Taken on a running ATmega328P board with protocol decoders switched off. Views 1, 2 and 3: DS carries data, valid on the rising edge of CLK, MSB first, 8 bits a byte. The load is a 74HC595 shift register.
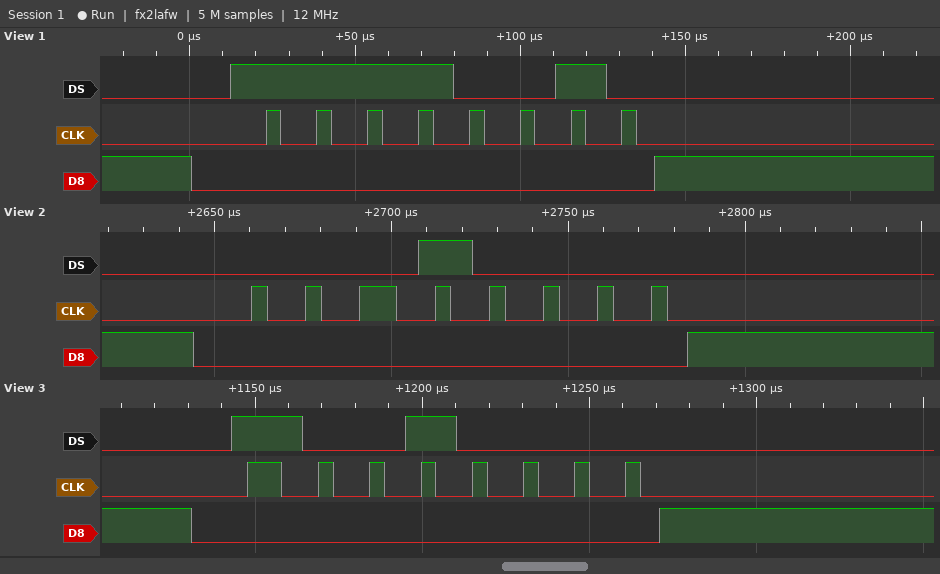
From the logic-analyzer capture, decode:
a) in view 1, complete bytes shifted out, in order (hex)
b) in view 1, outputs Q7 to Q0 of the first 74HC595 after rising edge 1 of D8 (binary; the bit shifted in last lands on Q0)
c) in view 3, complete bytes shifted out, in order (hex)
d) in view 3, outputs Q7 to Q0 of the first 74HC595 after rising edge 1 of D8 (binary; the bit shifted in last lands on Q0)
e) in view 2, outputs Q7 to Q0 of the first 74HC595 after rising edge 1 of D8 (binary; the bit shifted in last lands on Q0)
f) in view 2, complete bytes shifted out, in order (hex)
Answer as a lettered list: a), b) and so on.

a) F2
b) 11110010
c) 90
d) 10010000
e) 00010000
f) 10
